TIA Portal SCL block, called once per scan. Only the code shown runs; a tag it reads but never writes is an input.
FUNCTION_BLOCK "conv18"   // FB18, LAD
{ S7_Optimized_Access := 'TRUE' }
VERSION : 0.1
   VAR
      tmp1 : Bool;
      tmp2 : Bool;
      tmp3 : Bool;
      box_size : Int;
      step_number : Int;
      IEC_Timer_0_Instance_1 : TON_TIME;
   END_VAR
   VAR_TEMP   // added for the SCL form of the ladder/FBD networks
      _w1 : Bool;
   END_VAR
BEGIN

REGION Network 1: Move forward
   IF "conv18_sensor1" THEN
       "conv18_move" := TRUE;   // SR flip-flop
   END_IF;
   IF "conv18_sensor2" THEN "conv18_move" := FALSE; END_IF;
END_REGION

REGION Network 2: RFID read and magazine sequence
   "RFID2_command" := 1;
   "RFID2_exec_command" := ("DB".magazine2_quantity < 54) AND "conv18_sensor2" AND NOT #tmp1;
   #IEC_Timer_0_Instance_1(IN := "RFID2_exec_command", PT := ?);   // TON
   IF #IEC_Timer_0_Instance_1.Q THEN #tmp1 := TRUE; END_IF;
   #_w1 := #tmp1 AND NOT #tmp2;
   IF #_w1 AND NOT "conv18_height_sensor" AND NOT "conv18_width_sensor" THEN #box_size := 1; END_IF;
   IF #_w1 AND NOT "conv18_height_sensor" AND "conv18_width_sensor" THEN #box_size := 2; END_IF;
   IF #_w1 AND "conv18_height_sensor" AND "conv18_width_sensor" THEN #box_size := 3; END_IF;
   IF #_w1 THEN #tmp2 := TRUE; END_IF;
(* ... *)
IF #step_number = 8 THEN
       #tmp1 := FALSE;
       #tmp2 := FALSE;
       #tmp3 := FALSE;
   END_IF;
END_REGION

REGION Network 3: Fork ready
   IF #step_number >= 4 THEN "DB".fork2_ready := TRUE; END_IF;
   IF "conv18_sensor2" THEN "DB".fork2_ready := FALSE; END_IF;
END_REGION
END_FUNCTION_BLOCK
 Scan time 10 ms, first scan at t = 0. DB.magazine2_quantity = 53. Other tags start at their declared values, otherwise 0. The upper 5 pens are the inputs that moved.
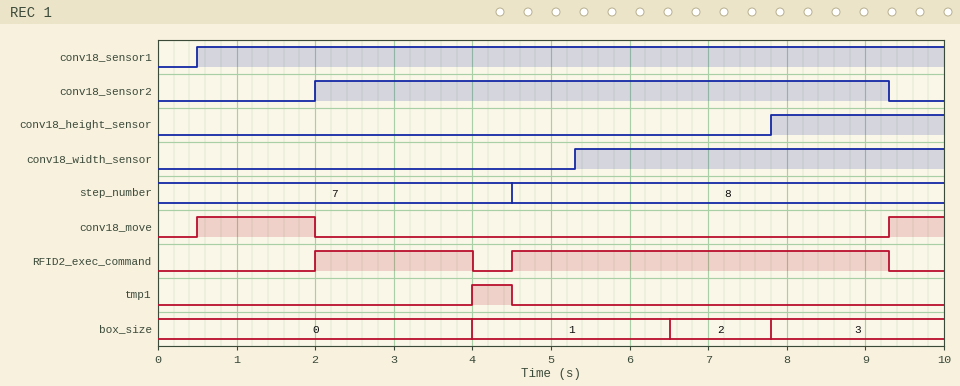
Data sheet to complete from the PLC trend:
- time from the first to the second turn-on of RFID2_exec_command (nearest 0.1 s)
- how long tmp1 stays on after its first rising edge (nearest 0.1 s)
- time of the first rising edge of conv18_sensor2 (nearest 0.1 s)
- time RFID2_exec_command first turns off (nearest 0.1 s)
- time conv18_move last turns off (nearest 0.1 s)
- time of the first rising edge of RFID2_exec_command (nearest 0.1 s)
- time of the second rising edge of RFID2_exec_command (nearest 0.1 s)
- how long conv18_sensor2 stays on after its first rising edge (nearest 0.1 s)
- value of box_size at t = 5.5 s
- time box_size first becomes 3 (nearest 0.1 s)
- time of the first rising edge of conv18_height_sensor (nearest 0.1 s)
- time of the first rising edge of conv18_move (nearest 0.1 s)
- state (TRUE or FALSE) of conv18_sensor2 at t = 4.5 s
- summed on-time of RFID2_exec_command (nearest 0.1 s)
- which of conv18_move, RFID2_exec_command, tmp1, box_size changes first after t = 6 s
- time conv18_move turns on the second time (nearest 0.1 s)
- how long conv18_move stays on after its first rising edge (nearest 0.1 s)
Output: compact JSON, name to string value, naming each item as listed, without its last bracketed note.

{"time from the first to the second turn-on of RFID2_exec_command": "2.5 s", "how long tmp1 stays on after its first rising edge": "0.5 s", "time of the first rising edge of conv18_sensor2": "2.0 s", "time RFID2_exec_command first turns off": "4.0 s", "time conv18_move last turns off": "2.0 s", "time of the first rising edge of RFID2_exec_command": "2.0 s", "time of the second rising edge of RFID2_exec_command": "4.5 s", "how long conv18_sensor2 stays on after its first rising edge": "7.3 s", "value of box_size at t = 5.5 s": "1", "time box_size first becomes 3": "7.8 s", "time of the first rising edge of conv18_height_sensor": "7.8 s", "time of the first rising edge of conv18_move": "0.5 s", "state (TRUE or FALSE) of conv18_sensor2 at t = 4.5 s": "TRUE", "summed on-time of RFID2_exec_command": "6.8 s", "which of conv18_move, RFID2_exec_command, tmp1, box_size changes first after t = 6 s": "box_size", "time conv18_move turns on the second time": "9.3 s", "how long conv18_move stays on after its first rising edge": "1.5 s"}
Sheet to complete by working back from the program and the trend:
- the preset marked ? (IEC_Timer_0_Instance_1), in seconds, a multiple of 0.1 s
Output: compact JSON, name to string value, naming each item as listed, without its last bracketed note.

{"the preset marked ? (IEC_Timer_0_Instance_1), in seconds, a multiple of 0.1 s": "2.0 s"}
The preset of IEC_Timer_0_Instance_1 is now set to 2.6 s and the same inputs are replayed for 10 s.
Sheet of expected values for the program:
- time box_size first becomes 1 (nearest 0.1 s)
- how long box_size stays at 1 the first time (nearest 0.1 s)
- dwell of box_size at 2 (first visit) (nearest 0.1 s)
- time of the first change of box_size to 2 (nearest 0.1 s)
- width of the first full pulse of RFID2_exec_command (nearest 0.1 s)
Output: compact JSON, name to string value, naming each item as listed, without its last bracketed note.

{"time box_size first becomes 1": "4.6 s", "how long box_size stays at 1 the first time": "0.7 s", "dwell of box_size at 2 (first visit)": "2.5 s", "time of the first change of box_size to 2": "5.3 s", "width of the first full pulse of RFID2_exec_command": "7.3 s"}
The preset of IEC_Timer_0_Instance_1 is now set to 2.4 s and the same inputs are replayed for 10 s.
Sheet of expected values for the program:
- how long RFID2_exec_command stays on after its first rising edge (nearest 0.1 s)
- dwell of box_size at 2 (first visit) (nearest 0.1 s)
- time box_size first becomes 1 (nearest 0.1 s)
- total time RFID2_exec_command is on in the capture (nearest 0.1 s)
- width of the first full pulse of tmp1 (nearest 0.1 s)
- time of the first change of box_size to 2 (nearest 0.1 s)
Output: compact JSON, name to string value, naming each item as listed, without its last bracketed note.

{"how long RFID2_exec_command stays on after its first rising edge": "2.4 s", "dwell of box_size at 2 (first visit)": "0.9 s", "time box_size first becomes 1": "4.4 s", "total time RFID2_exec_command is on in the capture": "7.2 s", "width of the first full pulse of tmp1": "0.1 s", "time of the first change of box_size to 2": "6.9 s"}
